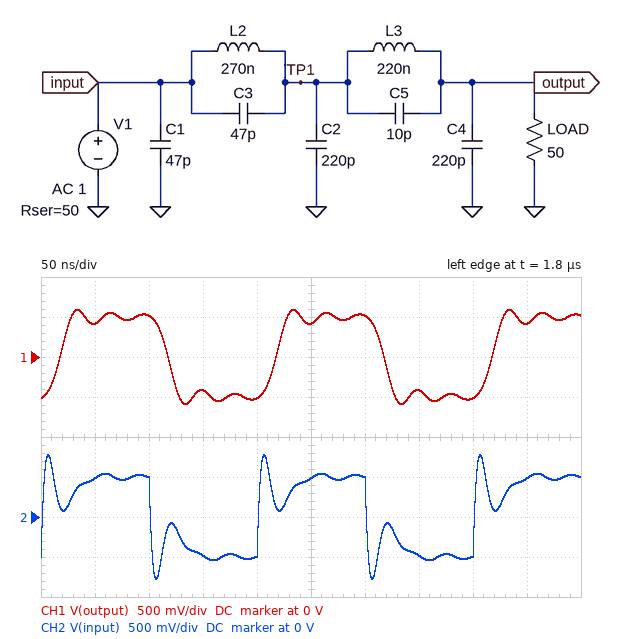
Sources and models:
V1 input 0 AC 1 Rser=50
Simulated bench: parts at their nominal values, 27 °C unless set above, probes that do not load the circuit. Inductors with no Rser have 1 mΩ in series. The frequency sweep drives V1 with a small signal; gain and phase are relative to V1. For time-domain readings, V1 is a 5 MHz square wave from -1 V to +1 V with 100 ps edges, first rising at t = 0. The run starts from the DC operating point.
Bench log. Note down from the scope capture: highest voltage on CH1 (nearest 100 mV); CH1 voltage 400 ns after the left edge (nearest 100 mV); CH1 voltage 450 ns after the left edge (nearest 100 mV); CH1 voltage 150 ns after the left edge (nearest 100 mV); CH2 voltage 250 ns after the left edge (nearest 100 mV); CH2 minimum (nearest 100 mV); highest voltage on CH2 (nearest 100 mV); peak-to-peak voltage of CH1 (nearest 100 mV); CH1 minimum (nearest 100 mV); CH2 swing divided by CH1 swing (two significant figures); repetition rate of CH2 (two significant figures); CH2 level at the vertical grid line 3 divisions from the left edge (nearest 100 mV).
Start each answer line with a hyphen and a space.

- 600 mV
- -500 mV
- 400 mV
- -400 mV
- 500 mV
- -800 mV
- 800 mV
- 1.2 V
- -600 mV
- 1.3
- 5.0 MHz
- -500 mV
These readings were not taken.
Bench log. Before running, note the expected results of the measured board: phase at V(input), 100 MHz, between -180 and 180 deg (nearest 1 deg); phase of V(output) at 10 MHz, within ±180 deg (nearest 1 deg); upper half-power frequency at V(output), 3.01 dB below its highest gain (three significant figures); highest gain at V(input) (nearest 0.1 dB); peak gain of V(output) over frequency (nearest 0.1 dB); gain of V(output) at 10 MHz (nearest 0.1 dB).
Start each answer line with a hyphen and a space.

- -68 deg
- -60 deg
- 33.2 MHz
- -0.3 dB
- -6.0 dB
- -6.7 dB
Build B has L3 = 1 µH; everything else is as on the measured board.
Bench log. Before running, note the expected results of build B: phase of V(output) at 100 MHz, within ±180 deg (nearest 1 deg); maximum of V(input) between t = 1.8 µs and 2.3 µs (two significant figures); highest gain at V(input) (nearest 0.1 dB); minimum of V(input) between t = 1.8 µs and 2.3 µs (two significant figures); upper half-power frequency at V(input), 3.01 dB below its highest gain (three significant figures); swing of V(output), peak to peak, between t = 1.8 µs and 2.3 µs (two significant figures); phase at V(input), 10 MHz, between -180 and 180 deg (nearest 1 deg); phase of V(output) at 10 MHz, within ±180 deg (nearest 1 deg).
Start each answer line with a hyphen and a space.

- -60 deg
- 870 mV
- 0 dB
- -870 mV
- 53.1 MHz
- 1.2 V
- 0 deg
- -98 deg
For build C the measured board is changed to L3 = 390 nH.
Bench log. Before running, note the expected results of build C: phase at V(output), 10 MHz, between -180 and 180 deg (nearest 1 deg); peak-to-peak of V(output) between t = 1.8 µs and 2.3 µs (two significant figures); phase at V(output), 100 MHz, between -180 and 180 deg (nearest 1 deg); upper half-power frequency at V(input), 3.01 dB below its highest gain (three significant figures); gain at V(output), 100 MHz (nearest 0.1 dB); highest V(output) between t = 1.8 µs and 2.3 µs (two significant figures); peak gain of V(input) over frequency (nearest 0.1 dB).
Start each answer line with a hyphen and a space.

- -67 deg
- 1.3 V
- -60 deg
- 53.4 MHz
- -61.6 dB
- 650 mV
- 0 dB
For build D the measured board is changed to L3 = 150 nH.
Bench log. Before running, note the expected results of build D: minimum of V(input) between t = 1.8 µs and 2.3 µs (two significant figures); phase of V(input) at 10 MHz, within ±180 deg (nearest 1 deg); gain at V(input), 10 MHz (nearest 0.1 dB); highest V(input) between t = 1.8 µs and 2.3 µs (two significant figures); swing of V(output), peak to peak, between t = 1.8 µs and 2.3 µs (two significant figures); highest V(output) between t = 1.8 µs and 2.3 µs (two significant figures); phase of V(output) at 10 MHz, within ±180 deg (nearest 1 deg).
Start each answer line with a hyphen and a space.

- -750 mV
- -6 deg
- -10.7 dB
- 750 mV
- 1.0 V
- 520 mV
- -57 deg
